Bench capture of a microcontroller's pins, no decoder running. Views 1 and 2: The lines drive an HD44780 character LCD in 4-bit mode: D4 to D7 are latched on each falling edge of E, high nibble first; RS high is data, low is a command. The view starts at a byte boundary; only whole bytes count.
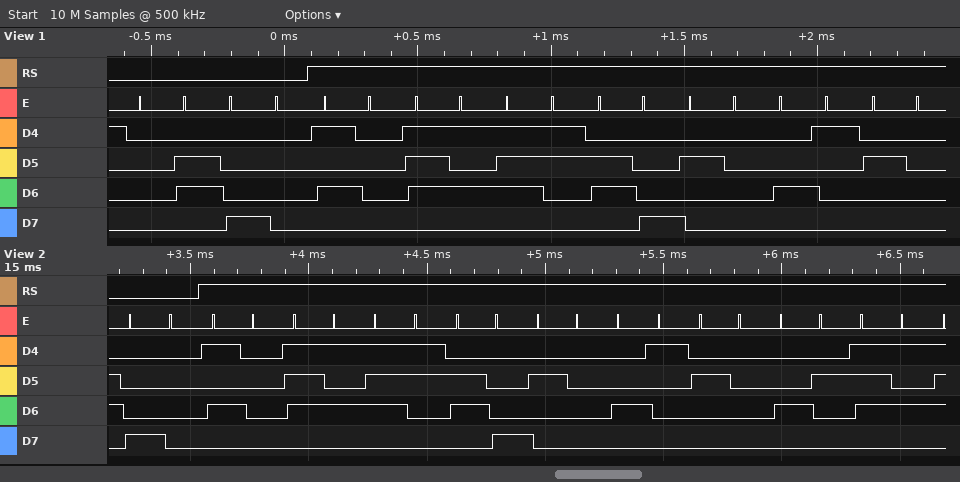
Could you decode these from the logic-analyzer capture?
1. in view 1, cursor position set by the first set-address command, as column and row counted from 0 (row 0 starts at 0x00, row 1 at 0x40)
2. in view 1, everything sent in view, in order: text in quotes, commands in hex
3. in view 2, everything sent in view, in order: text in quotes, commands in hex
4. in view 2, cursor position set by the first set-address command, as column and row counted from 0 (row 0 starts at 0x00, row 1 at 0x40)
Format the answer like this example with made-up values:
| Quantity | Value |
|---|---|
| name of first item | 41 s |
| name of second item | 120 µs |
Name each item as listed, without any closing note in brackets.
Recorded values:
| Quantity | Value |
|---|---|
| in view 1, cursor position set by the first set-address command, as column and row counted from 0 | column 0, row 0 |
| in view 1, everything sent in view, in order: text in quotes, commands in hex | 0x06 0x80 "Push A " |
| in view 2, everything sent in view, in order: text in quotes, commands in hex | 0x80 "Push A Bu" |
| in view 2, cursor position set by the first set-address command, as column and row counted from 0 | column 0, row 0 |
